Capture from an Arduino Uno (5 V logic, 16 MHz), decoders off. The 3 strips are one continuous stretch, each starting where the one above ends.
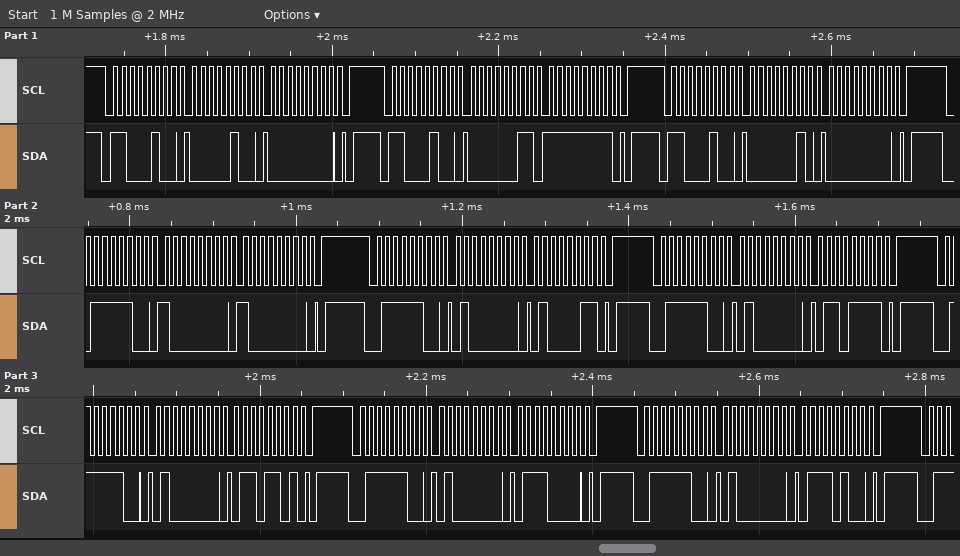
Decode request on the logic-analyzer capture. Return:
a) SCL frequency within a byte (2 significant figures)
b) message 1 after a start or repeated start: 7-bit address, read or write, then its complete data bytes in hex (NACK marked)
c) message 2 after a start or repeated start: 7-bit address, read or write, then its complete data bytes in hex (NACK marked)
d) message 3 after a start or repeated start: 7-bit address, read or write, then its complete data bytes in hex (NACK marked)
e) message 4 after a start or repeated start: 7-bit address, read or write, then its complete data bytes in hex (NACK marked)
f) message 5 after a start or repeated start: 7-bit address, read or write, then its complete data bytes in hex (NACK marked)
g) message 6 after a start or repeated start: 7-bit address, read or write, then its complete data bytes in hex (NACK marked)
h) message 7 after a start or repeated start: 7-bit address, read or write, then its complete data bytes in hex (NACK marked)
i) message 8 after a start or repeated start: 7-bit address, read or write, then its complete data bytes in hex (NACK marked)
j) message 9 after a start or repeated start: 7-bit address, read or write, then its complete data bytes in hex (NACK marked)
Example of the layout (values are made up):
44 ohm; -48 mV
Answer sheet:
100 kHz; 0x62 write: 04 00; 0x62 write: 03 FF; 0x62 write: 02 00; 0x3E write: 80 80; 0x3E write: 40 43; 0x3E write: 40 6F; 0x3E write: 40 6D; 0x3E write: 40 70; 0x3E write: 40 74
